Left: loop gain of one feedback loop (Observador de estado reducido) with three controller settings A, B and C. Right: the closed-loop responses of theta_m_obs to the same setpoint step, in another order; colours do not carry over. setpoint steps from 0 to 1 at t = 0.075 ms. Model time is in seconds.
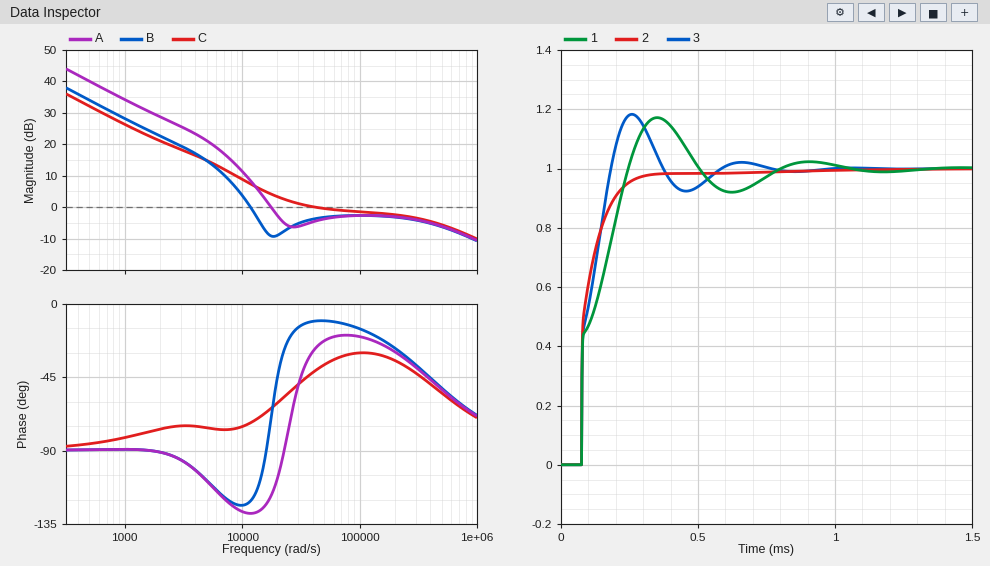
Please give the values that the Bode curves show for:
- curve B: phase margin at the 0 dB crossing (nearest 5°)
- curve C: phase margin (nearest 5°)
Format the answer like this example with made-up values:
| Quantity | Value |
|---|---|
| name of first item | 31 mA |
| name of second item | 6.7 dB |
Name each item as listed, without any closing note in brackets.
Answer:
| Quantity | Value |
|---|---|
| curve B: phase margin at the 0 dB crossing | 60° |
| curve C: phase margin | 140° |
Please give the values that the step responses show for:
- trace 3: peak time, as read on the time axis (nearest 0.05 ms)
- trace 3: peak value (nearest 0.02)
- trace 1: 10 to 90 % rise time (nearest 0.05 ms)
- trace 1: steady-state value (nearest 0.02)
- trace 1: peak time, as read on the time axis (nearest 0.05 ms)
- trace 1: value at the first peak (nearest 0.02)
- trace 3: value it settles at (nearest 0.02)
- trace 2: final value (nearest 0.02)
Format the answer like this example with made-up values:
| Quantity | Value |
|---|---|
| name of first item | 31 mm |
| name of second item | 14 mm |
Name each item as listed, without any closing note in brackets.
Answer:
| Quantity | Value |
|---|---|
| trace 3: peak time, as read on the time axis | 0.25 ms |
| trace 3: peak value | 1.18 |
| trace 1: 10 to 90 % rise time | 0.15 ms |
| trace 1: steady-state value | 1.00 |
| trace 1: peak time, as read on the time axis | 0.35 ms |
| trace 1: value at the first peak | 1.18 |
| trace 3: value it settles at | 1.00 |
| trace 2: final value | 1.00 |
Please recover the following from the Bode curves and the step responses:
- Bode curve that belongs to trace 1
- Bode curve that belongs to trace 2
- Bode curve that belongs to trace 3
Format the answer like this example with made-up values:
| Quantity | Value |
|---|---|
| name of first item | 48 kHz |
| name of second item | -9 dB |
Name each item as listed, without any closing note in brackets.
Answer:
| Quantity | Value |
|---|---|
| Bode curve that belongs to trace 1 | B |
| Bode curve that belongs to trace 2 | C |
| Bode curve that belongs to trace 3 | A |
